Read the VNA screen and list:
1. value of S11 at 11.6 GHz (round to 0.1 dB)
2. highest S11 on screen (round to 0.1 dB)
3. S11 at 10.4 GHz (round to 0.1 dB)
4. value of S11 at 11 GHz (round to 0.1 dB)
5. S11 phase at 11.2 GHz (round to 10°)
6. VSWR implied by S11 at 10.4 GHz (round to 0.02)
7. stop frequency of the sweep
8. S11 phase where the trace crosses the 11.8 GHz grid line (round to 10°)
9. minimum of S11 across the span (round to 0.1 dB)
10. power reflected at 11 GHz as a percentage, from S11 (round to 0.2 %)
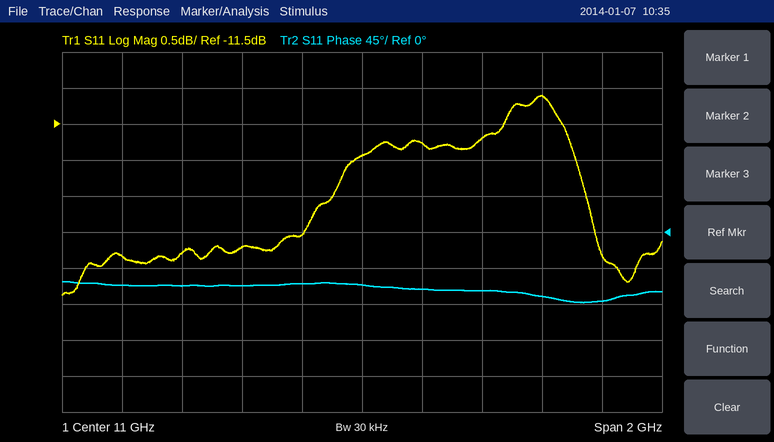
-11.1 dB
-11.1 dB
-13.3 dB
-11.9 dB
-70°
1.56
12 GHz
-90°
-13.9 dB
6.4 %
